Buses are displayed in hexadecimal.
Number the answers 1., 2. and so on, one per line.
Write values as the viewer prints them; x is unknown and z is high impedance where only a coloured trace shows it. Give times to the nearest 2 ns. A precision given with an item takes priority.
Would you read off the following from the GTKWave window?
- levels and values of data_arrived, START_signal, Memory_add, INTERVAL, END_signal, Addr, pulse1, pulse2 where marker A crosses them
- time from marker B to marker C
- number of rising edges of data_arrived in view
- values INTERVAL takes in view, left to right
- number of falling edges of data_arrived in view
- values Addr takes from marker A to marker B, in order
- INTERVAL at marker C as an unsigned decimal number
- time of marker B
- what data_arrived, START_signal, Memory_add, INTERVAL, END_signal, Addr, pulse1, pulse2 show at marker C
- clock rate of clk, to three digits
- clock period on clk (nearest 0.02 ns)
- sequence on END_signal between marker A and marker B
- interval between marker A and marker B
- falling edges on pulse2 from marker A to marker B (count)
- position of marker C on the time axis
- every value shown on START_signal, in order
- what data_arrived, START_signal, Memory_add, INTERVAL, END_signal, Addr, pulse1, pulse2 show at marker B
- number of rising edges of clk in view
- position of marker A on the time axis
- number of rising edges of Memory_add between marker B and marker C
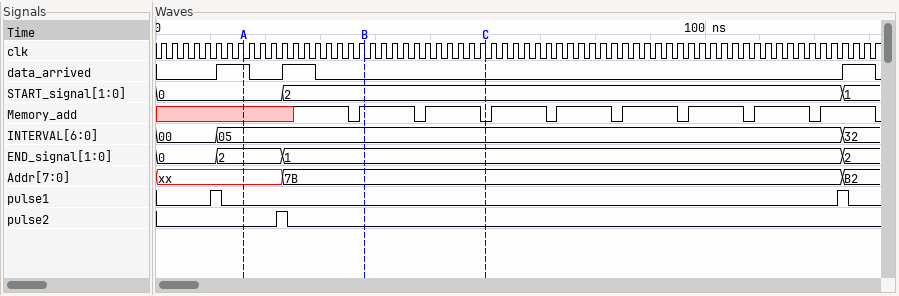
1. data_arrived=1, START_signal=0, Memory_add=x, INTERVAL=05, END_signal=2, Addr=xx, pulse1=0, pulse2=0
2. 22 ns
3. 3
4. 00, 05, 32
5. 3
6. xx, 7B
7. 5
8. 38 ns
9. data_arrived=0, START_signal=2, Memory_add=0, INTERVAL=05, END_signal=1, Addr=7B, pulse1=0, pulse2=0
10. 500 MHz
11. 2 ns
12. 2, 1
13. 22 ns
14. 1
15. 60 ns
16. 0, 2, 1
17. data_arrived=0, START_signal=2, Memory_add=1, INTERVAL=05, END_signal=1, Addr=7B, pulse1=0, pulse2=0
18. 66
19. 16 ns
20. 1
